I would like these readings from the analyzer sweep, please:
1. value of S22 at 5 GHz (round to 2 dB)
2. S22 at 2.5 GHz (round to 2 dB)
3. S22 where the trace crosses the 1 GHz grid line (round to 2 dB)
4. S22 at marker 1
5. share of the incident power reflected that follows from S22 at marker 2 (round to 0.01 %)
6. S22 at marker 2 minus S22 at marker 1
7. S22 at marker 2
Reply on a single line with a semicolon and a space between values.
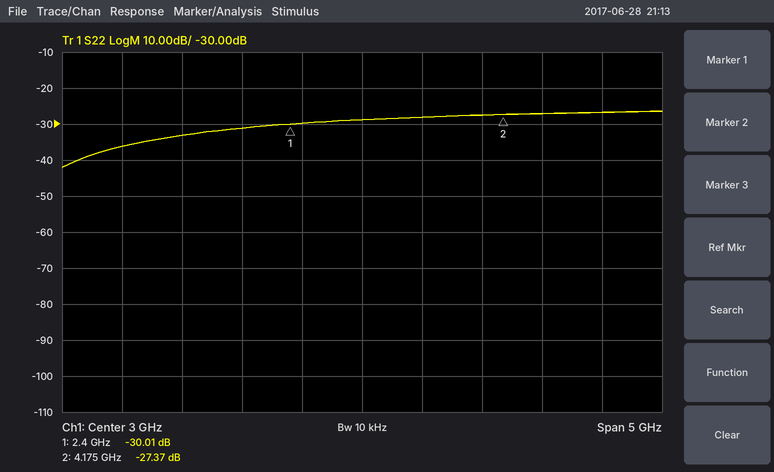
-26 dB; -30 dB; -36 dB; -30.01 dB; 0.18 %; 2.64 dB; -27.37 dB
